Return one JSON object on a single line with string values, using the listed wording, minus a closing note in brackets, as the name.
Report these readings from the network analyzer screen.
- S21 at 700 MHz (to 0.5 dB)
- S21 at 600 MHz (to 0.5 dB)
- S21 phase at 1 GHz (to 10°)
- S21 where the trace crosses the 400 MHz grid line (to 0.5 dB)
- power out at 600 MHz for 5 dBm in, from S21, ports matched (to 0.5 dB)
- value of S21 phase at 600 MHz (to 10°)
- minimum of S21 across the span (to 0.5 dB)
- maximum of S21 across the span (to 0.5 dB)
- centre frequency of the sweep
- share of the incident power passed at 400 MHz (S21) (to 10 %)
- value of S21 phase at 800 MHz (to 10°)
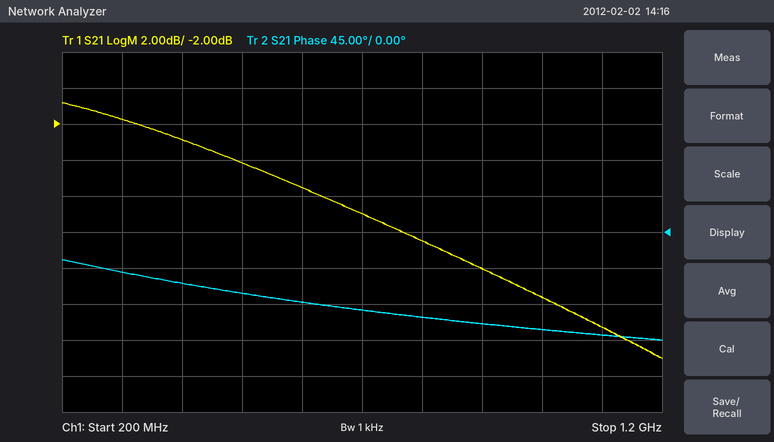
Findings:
{"S21 at 700 MHz": "-7.0 dB", "S21 at 600 MHz": "-5.5 dB", "S21 phase at 1 GHz": "-120°", "S21 where the trace crosses the 400 MHz grid line": "-3.0 dB", "power out at 600 MHz for 5 dBm in, from S21, ports matched": "-0.5 dBm", "value of S21 phase at 600 MHz": "-90°", "minimum of S21 across the span": "-15.0 dB", "maximum of S21 across the span": "-1.0 dB", "centre frequency of the sweep": "700 MHz", "share of the incident power passed at 400 MHz (S21)": "50 %", "value of S21 phase at 800 MHz": "-110°"}
